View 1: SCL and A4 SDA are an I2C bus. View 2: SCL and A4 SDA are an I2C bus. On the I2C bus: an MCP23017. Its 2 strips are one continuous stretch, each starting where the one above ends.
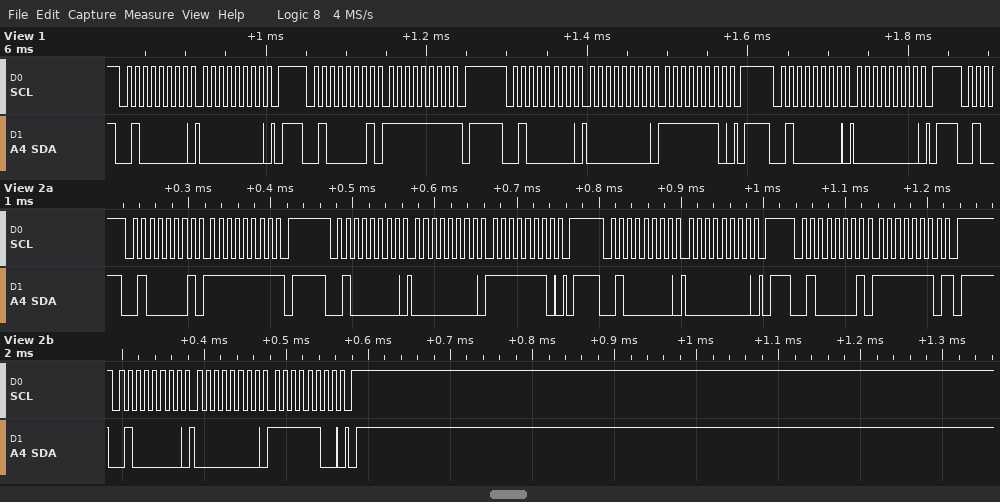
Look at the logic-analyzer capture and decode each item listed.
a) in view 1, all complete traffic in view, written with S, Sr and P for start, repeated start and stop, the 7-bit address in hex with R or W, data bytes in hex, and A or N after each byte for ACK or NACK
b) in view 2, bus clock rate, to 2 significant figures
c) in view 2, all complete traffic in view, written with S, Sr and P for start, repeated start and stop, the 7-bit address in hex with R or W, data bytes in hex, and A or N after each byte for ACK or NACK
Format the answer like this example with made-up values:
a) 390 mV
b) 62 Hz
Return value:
a) S 20W A 00 A P S 20R A FF N P S 20W A 00 A FE A P S 20W A 00 A P
b) 100 kHz
c) S 20R A FF N P S 20W A 00 A FE A P S 20W A 00 A P S 20R A FE N P S 20W A 00 A FC A P
